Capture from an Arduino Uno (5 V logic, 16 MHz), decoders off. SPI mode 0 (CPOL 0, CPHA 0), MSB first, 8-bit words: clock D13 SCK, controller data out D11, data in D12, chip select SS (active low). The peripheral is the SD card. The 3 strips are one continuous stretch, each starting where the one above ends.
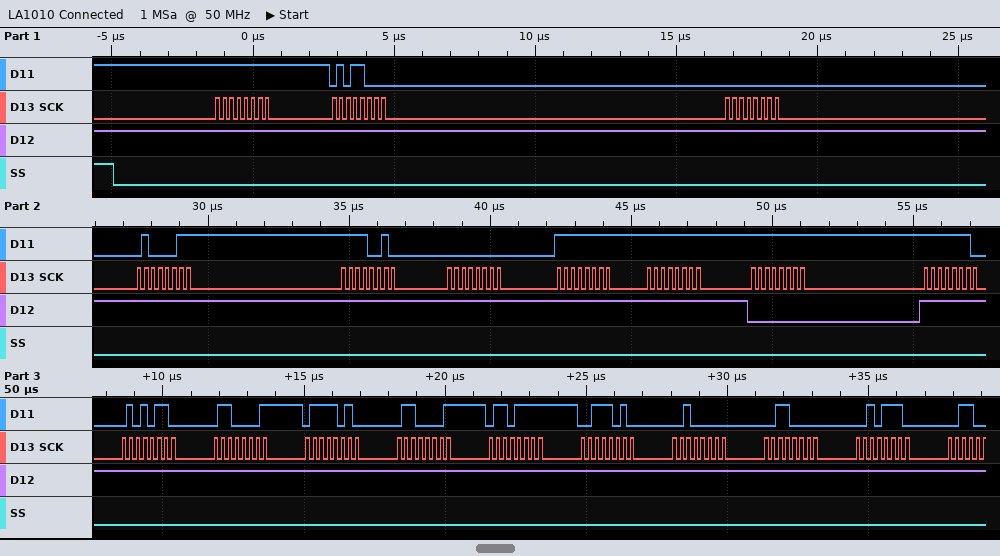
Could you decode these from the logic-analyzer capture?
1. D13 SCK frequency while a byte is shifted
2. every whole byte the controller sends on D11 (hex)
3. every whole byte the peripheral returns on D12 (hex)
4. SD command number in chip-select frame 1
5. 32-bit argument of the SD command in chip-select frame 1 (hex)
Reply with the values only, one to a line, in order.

4 MHz
0xFF 0x58 0x00 0x43 0xF2 0x00 0xFF 0xFF 0xFF 0xFE 0x56 0x61 0x7A 0x61 0x6F 0x3A 0x20 0x30 0x2E
0xFF 0xFF 0xFF 0xFF 0xFF 0xFF 0xFF 0xFF 0x00 0xFF 0xFF 0xFF 0xFF 0xFF 0xFF 0xFF 0xFF 0xFF 0xFF
CMD24
0x0043F200
